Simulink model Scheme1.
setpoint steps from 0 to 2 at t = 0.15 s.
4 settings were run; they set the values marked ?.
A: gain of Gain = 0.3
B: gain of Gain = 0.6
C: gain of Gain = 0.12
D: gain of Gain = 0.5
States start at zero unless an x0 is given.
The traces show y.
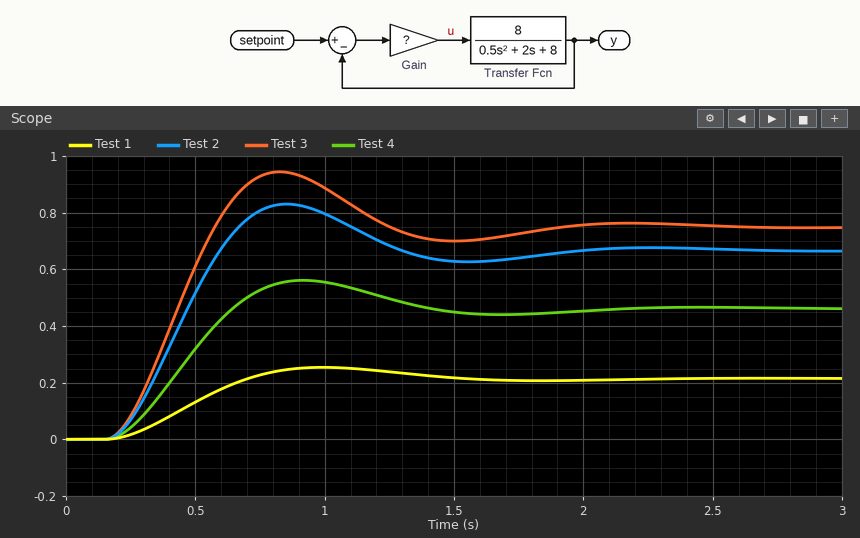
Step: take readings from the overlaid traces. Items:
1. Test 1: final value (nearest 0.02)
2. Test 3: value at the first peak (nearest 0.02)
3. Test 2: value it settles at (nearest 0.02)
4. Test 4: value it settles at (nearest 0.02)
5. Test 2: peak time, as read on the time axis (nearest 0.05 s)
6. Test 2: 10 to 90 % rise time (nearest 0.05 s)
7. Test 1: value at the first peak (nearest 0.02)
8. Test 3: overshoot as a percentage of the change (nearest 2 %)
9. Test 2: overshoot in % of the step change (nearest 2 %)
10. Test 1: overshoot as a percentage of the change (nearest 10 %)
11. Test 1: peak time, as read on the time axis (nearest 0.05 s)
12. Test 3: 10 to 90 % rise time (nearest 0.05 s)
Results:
0.22
0.94
0.66
0.46
0.85 s
0.30 s
0.26
26 %
24 %
20 %
1.00 s
0.30 s
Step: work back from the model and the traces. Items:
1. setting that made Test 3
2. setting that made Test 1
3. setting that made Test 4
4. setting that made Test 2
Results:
B
C
A
D
